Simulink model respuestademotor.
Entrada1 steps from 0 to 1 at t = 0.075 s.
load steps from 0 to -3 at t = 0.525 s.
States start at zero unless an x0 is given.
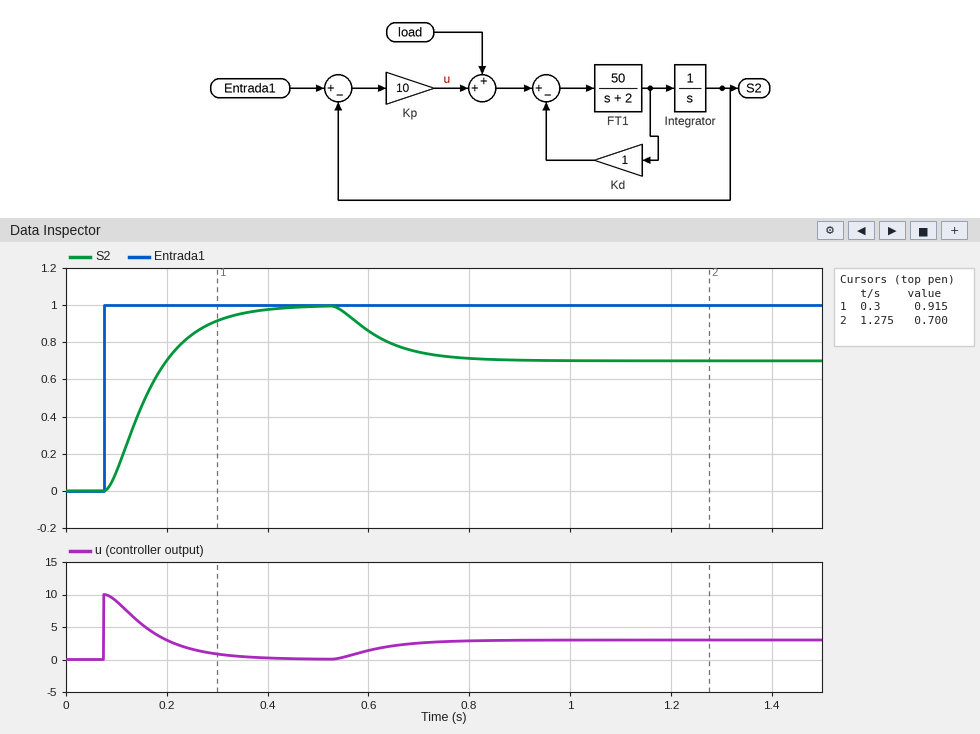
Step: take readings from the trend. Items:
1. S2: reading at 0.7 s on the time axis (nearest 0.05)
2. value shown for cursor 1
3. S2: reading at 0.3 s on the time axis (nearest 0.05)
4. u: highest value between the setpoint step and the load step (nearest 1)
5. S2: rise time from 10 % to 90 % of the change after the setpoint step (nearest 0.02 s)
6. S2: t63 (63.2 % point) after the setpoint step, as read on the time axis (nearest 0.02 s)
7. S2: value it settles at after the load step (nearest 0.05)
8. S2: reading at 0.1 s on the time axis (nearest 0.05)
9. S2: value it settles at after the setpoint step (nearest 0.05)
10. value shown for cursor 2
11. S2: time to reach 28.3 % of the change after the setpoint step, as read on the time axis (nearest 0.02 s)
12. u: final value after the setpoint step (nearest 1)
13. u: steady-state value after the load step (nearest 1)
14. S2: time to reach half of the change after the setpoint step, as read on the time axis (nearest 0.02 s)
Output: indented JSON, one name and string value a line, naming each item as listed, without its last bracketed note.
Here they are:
{
  "S2: reading at 0.7 s on the time axis": "0.75",
  "value shown for cursor 1": "0.915",
  "S2: reading at 0.3 s on the time axis": "0.90",
  "u: highest value between the setpoint step and the load step": "10",
  "S2: rise time from 10 % to 90 % of the change after the setpoint step": "0.18 s",
  "S2: t63 (63.2 % point) after the setpoint step, as read on the time axis": "0.18 s",
  "S2: value it settles at after the load step": "0.70",
  "S2: reading at 0.1 s on the time axis": "0.10",
  "S2: value it settles at after the setpoint step": "1.00",
  "value shown for cursor 2": "0.700",
  "S2: time to reach 28.3 % of the change after the setpoint step, as read on the time axis": "0.12 s",
  "u: final value after the setpoint step": "0",
  "u: steady-state value after the load step": "3",
  "S2: time to reach half of the change after the setpoint step, as read on the time axis": "0.16 s"
}
